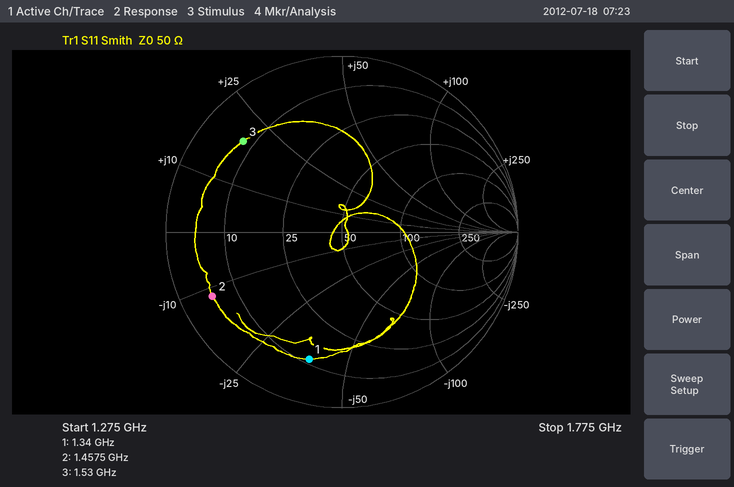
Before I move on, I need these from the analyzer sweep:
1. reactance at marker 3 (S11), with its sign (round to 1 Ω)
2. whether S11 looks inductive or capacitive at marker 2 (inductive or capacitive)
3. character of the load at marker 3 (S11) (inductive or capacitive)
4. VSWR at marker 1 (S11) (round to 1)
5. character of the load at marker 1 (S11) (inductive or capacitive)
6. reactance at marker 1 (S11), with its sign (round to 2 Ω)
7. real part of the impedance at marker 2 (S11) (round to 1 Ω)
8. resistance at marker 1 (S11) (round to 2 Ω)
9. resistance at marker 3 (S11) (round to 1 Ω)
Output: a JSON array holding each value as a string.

["+19 Ω", "capacitive", "inductive", "7", "capacitive", "-38 Ω", "5 Ω", "12 Ω", "8 Ω"]
